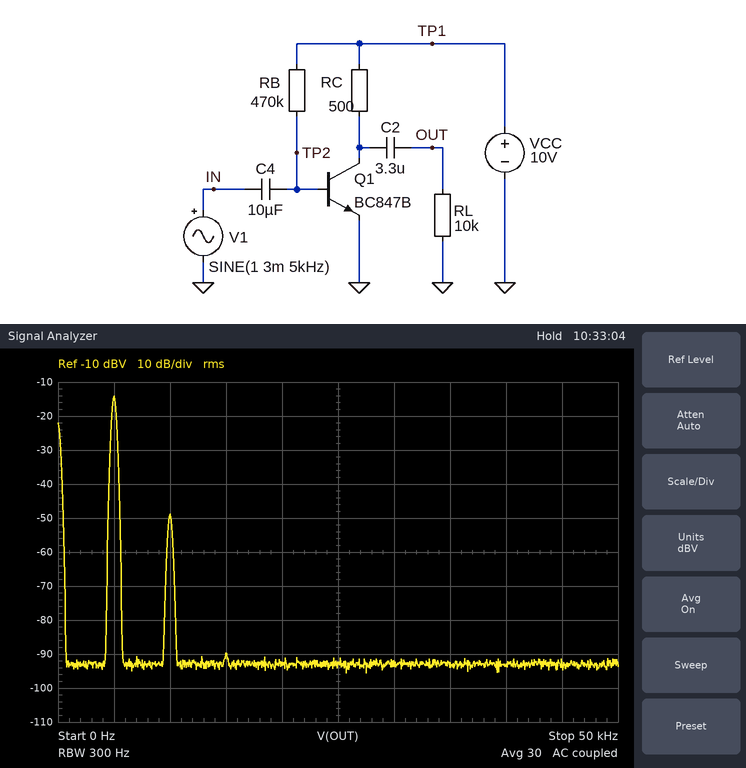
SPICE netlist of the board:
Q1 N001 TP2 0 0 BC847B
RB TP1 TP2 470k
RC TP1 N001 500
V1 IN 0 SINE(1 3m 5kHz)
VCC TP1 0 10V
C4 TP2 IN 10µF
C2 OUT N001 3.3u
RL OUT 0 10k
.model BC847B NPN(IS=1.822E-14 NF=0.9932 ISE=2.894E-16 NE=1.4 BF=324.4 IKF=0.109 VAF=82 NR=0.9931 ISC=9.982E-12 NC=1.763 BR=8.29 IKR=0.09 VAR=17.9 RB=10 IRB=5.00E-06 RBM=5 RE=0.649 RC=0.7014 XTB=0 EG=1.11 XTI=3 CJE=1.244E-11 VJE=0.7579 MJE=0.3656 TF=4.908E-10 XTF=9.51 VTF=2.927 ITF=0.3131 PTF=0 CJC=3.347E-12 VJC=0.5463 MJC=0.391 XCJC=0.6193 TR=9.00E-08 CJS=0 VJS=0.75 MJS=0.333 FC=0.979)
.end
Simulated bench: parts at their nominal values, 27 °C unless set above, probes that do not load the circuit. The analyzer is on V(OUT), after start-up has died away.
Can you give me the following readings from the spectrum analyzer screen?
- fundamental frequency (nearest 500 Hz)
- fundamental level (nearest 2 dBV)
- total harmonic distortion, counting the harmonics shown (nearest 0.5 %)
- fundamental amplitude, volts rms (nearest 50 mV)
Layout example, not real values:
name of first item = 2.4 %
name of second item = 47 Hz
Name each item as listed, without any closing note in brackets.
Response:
fundamental frequency = 5.0 kHz
fundamental level = -14 dBV
total harmonic distortion, counting the harmonics shown = 2.0 %
fundamental amplitude, volts rms = 200 mV
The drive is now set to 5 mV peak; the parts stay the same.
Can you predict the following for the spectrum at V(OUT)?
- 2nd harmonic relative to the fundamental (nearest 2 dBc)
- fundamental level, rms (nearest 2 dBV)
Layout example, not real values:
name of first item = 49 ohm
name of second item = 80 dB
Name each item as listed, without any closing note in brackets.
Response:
2nd harmonic relative to the fundamental = -30 dBc
fundamental level, rms = -10 dBV
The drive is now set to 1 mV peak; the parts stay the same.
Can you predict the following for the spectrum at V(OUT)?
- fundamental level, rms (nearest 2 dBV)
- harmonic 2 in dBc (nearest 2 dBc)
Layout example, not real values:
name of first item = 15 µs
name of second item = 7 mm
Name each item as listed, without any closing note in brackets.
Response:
fundamental level, rms = -24 dBV
harmonic 2 in dBc = -44 dBc
